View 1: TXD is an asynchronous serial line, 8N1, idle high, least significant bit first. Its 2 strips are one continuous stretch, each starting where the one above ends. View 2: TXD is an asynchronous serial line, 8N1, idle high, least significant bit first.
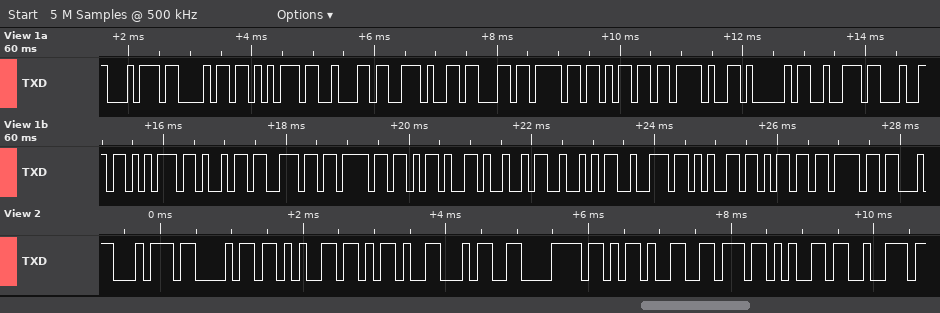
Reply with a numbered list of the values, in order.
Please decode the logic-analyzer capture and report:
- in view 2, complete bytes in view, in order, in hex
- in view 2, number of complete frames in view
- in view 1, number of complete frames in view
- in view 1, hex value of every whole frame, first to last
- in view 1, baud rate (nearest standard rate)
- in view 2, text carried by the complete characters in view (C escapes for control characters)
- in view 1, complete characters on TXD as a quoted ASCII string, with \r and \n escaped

1. 74 68 65 2D 34 78 2D 76 65 72
2. 10
3. 23
4. 0x74 0x68 0x75 0x62 0x2E 0x63 0x6F 0x6D 0x2F 0x41 0x72 0x64 0x75 0x69 0x6E 0x6F 0x2D 0x49 0x52 0x72 0x65 0x6D 0x6F
5. 9600 baud
6. "the-4x-ver"
7. "thub.com/Arduino-IRremo"
